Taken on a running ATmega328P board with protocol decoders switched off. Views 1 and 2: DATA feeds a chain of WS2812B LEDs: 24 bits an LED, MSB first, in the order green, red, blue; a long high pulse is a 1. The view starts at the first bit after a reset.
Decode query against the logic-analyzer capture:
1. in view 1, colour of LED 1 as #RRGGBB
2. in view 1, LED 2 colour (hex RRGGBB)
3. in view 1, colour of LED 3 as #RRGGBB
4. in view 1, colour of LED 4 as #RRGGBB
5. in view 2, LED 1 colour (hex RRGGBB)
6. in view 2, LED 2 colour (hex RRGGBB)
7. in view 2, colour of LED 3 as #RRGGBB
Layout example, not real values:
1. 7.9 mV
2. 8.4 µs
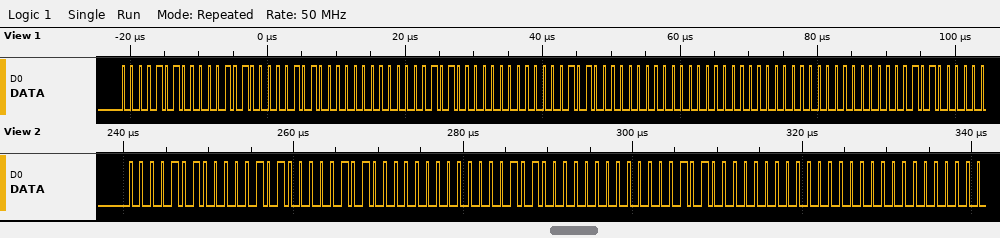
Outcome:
1. #0A0A0A
2. #0A0000
3. #000A00
4. #00000A
5. #0A0A0A
6. #0A0000
7. #000A00
